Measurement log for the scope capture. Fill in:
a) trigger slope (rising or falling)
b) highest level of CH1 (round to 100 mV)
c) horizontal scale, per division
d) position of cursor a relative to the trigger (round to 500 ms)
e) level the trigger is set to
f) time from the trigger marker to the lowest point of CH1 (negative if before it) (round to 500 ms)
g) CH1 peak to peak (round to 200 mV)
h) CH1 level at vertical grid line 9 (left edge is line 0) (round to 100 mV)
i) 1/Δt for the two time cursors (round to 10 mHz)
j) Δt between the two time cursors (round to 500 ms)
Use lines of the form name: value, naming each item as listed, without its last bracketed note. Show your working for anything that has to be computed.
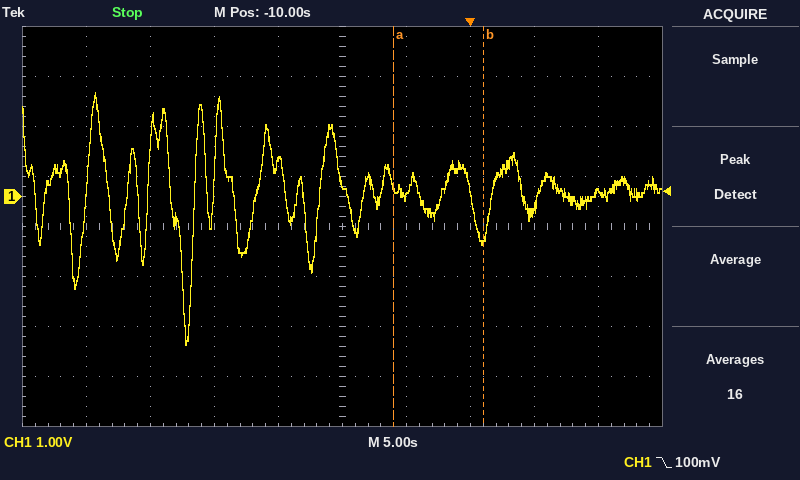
trigger slope: falling
highest level of CH1: 2.1 V
horizontal scale, per division: 5 s
position of cursor a relative to the trigger: -6.0 s
level the trigger is set to: 100 mV
time from the trigger marker to the lowest point of CH1 (negative if before it): -22.0 s
CH1 peak to peak: 5.0 V
CH1 level at vertical grid line 9 (left edge is line 0): 100 mV
1/Δt for the two time cursors: 1 / 7.0 s ≈ 140 mHz
Δt between the two time cursors: 7.0 s
